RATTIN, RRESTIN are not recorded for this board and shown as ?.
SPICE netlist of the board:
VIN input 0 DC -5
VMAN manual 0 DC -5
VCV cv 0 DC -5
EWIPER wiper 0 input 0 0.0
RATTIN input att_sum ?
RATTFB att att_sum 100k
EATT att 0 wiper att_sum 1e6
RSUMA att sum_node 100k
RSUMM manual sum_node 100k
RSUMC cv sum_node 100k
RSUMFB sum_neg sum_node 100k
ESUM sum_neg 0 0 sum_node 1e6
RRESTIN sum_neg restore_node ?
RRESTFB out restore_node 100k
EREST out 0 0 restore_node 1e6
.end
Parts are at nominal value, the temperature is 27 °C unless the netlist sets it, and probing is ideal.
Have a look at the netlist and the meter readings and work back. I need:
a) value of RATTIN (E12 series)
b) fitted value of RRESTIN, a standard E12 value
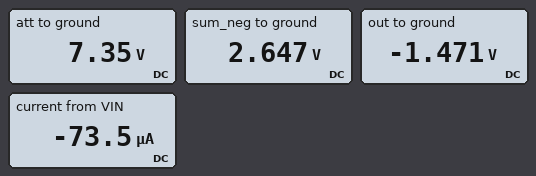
68 kΩ
180 kΩ
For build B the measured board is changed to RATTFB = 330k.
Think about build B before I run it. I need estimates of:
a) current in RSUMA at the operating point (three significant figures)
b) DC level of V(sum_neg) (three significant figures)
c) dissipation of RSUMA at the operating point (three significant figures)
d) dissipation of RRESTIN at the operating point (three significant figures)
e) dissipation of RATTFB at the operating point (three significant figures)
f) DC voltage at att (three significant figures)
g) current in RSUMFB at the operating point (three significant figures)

243 µA
-14.3 V
5.89 mW
1.13 mW
1.78 mW
24.3 V
143 µA
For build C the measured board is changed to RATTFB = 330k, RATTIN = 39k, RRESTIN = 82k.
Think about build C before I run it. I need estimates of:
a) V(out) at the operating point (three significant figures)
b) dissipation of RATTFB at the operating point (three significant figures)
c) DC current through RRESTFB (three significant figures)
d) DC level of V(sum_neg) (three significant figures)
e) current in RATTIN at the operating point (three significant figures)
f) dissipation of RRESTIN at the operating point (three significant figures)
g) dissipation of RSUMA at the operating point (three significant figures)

39.4 V
5.42 mW
394 µA
-32.3 V
128 µA
12.7 mW
17.9 mW
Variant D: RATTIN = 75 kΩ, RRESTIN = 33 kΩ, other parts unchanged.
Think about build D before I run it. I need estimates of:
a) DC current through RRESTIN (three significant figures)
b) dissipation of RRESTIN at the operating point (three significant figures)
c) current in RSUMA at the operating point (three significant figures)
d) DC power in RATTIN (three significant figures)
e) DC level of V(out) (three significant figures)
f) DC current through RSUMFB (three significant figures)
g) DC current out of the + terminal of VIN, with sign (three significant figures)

101 µA
337 µW
66.7 µA
333 µW
-10.1 V
33.3 µA
-66.7 µA
